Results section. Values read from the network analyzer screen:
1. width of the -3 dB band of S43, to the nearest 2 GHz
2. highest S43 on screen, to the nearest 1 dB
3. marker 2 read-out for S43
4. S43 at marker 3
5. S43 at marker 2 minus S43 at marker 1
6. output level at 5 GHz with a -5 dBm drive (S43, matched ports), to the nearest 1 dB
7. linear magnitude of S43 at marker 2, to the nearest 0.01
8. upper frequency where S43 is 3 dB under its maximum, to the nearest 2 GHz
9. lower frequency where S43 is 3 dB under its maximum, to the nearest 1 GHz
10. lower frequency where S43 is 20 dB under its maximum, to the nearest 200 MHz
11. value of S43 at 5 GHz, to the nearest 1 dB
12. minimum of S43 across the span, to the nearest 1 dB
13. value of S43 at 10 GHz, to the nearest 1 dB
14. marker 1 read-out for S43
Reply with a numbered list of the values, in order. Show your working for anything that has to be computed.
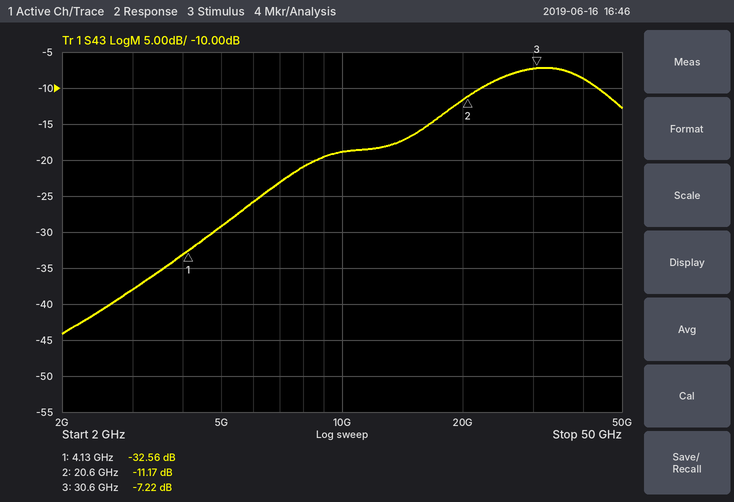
1. 44 GHz − 22 GHz = 22 GHz
2. -7 dB
3. -11.17 dB
4. -7.22 dB
5. -11.17 − (-32.56) = 21.39 dB
6. -5 dBm + (-29 dB) = -34 dBm
7. 10^(-11.17/20) ≈ 0.28
8. 44 GHz
9. 22 GHz
10. 5.6 GHz
11. -29 dB
12. -44 dB
13. -19 dB
14. -32.56 dB
